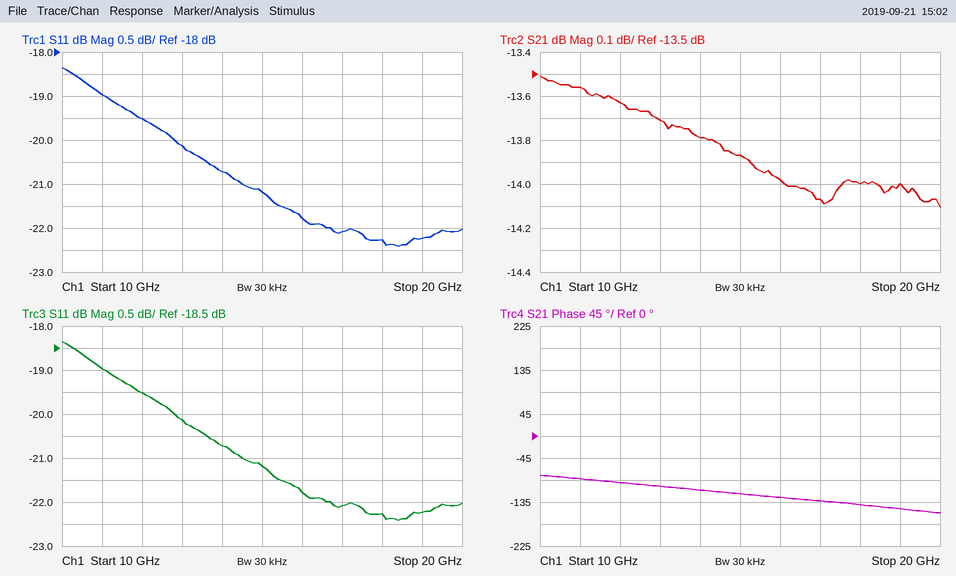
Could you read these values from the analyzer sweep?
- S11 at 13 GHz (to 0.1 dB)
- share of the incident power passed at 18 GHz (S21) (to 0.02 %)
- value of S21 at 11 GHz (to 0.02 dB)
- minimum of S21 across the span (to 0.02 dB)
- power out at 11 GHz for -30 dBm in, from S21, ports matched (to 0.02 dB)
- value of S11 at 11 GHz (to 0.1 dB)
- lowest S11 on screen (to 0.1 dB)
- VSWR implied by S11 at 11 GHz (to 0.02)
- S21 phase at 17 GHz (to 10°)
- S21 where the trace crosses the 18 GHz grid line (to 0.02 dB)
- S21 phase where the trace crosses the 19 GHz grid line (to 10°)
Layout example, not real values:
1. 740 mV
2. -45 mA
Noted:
1. -20.1 dB
2. 3.98 %
3. -13.56 dB
4. -14.10 dB
5. -43.56 dBm
6. -19.0 dB
7. -22.4 dB
8. 1.26
9. -130°
10. -14.00 dB
11. -150°
